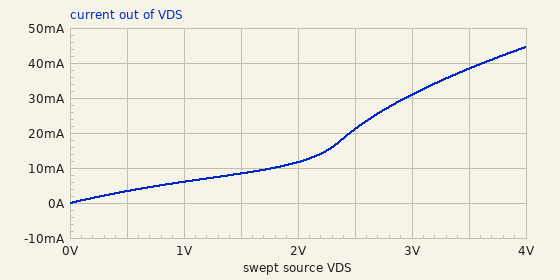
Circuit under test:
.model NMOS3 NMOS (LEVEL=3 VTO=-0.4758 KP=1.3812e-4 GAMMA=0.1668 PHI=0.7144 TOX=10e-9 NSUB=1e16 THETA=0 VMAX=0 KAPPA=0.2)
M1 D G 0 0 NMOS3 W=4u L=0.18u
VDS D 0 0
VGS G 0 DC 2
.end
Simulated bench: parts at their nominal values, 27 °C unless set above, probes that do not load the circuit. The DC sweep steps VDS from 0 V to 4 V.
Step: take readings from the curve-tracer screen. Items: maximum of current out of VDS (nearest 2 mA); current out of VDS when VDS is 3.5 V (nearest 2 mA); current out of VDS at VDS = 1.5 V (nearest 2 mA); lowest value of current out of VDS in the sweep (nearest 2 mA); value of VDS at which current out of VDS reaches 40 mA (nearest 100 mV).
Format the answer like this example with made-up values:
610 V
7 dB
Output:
44 mA
38 mA
8 mA
0 A
3.6 V
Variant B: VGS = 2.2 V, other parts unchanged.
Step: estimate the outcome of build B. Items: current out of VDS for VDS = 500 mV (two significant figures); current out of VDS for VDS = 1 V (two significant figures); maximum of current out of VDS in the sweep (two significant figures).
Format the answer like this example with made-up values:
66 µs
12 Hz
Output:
3.7 mA
6.7 mA
50 mA
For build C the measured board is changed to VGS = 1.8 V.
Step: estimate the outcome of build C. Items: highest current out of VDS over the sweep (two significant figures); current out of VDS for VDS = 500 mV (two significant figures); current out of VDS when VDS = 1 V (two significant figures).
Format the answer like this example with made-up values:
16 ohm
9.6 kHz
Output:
39 mA
3.1 mA
5.5 mA
